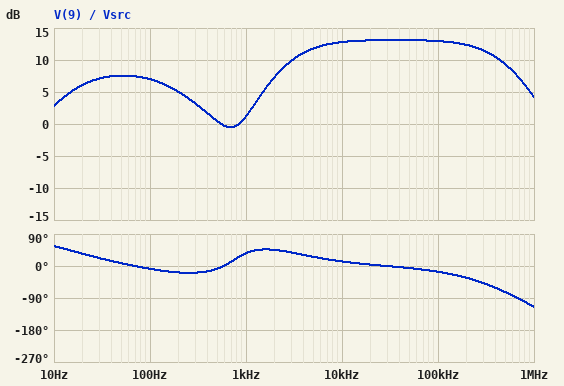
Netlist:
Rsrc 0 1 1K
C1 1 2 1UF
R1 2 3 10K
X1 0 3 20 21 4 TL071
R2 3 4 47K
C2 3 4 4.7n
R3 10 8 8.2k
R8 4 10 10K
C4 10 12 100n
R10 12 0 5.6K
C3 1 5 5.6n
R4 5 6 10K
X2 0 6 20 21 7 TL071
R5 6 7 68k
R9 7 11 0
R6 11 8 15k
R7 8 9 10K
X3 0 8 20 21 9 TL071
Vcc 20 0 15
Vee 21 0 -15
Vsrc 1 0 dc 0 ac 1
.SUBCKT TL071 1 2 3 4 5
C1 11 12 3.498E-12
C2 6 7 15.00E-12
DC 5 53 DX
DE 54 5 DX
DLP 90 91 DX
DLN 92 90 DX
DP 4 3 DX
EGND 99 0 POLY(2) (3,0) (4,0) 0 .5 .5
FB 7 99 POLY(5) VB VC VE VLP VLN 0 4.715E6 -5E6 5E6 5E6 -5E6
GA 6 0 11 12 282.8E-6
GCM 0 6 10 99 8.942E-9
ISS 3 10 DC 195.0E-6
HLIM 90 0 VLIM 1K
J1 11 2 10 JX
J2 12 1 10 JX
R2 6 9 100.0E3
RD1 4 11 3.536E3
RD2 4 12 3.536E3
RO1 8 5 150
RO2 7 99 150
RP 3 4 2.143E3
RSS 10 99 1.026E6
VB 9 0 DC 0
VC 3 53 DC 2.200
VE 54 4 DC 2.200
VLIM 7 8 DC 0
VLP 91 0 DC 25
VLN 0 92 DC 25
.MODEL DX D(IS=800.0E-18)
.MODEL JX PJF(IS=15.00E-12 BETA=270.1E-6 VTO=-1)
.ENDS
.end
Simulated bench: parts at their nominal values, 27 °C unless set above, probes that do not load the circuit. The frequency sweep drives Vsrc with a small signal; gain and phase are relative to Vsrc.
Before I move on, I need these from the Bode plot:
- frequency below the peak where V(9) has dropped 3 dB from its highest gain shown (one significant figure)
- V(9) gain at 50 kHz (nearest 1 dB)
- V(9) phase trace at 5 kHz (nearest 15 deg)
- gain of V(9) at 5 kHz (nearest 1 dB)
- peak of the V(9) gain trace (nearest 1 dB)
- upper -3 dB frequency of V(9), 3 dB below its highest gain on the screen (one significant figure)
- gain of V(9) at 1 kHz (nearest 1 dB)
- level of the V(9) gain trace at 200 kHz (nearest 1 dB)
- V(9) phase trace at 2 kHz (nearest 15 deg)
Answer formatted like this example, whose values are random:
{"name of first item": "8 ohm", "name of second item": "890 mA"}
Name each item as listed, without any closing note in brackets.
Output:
{"frequency below the peak where V(9) has dropped 3 dB from its highest gain shown": "3 kHz", "V(9) gain at 50 kHz": "13 dB", "V(9) phase trace at 5 kHz": "30 deg", "gain of V(9) at 5 kHz": "12 dB", "peak of the V(9) gain trace": "13 dB", "upper -3 dB frequency of V(9), 3 dB below its highest gain on the screen": "400 kHz", "gain of V(9) at 1 kHz": "1 dB", "level of the V(9) gain trace at 200 kHz": "12 dB", "V(9) phase trace at 2 kHz": "45 deg"}
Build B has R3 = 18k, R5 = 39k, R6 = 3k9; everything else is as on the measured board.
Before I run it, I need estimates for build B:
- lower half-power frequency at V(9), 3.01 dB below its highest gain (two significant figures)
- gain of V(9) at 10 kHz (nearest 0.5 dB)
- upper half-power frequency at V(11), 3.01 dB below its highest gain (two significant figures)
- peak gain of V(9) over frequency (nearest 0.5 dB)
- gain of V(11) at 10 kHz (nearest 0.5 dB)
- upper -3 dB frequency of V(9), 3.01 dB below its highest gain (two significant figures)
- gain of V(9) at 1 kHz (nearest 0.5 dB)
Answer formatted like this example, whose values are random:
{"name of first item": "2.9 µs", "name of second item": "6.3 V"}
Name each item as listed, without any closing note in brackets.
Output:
{"lower half-power frequency at V(9), 3.01 dB below its highest gain": "2.9 kHz", "gain of V(9) at 10 kHz": "19.5 dB", "upper half-power frequency at V(11), 3.01 dB below its highest gain": "750 kHz", "peak gain of V(9) over frequency": "20.0 dB", "gain of V(11) at 10 kHz": "11.5 dB", "upper -3 dB frequency of V(9), 3.01 dB below its highest gain": "550 kHz", "gain of V(9) at 1 kHz": "9.5 dB"}
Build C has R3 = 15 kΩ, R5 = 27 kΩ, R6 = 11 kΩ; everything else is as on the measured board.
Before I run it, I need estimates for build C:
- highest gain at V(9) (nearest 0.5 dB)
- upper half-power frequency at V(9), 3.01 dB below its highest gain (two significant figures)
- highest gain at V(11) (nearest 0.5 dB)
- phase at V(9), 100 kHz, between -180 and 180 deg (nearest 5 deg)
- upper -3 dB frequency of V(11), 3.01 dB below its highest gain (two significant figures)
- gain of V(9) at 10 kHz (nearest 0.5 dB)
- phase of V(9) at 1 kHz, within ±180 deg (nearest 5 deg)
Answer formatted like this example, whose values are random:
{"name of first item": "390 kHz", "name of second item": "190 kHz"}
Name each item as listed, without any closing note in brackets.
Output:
{"highest gain at V(9)": "8.0 dB", "upper half-power frequency at V(9), 3.01 dB below its highest gain": "840 kHz", "highest gain at V(11)": "8.5 dB", "phase at V(9), 100 kHz, between -180 and 180 deg": "-10 deg", "upper -3 dB frequency of V(11), 3.01 dB below its highest gain": "1.0 MHz", "gain of V(9) at 10 kHz": "7.5 dB", "phase of V(9) at 1 kHz, within ±180 deg": "30 deg"}
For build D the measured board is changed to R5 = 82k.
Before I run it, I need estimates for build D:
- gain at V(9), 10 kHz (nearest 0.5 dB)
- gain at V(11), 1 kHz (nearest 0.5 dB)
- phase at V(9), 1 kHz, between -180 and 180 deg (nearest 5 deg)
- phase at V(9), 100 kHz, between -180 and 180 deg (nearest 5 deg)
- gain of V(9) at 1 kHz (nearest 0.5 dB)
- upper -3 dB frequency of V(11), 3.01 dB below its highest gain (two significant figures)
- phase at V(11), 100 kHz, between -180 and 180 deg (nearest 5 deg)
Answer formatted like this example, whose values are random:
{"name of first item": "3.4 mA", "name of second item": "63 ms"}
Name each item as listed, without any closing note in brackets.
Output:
{"gain at V(9), 10 kHz": "14.5 dB", "gain at V(11), 1 kHz": "8.5 dB", "phase at V(9), 1 kHz, between -180 and 180 deg": "45 deg", "phase at V(9), 100 kHz, between -180 and 180 deg": "-20 deg", "gain of V(9) at 1 kHz": "3.0 dB", "upper -3 dB frequency of V(11), 3.01 dB below its highest gain": "380 kHz", "phase at V(11), 100 kHz, between -180 and 180 deg": "165 deg"}
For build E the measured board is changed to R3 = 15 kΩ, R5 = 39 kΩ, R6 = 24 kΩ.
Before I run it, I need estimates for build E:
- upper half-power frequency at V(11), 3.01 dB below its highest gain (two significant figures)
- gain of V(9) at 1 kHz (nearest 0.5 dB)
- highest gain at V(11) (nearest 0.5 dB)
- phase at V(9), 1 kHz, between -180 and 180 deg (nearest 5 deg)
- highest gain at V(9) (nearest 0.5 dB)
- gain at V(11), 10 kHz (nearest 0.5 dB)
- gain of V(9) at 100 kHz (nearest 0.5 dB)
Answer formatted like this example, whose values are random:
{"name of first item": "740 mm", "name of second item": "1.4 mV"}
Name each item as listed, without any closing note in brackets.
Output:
{"upper half-power frequency at V(11), 3.01 dB below its highest gain": "790 kHz", "gain of V(9) at 1 kHz": "-7.0 dB", "highest gain at V(11)": "12.0 dB", "phase at V(9), 1 kHz, between -180 and 180 deg": "5 deg", "highest gain at V(9)": "4.5 dB", "gain at V(11), 10 kHz": "11.5 dB", "gain of V(9) at 100 kHz": "4.0 dB"}
